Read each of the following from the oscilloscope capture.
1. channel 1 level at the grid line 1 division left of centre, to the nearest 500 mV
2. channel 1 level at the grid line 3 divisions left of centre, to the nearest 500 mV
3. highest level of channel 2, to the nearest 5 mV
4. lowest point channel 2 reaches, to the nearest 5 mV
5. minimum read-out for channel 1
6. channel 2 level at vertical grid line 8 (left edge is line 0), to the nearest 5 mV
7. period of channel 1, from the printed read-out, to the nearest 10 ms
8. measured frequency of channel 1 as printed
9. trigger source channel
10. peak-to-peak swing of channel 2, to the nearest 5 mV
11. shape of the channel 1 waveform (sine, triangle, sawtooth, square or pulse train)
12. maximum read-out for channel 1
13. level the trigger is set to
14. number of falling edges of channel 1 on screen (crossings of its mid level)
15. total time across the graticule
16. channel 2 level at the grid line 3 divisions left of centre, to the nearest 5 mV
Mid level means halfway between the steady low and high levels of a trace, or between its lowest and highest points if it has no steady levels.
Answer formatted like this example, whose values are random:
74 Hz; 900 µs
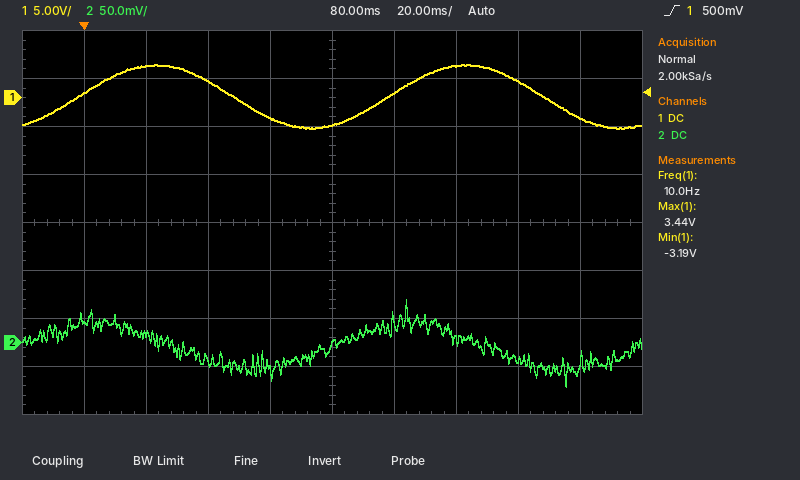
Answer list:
-2.0 V; 3.5 V; 45 mV; -45 mV; -3.19 V; -20 mV; 100 ms; 10.0 Hz; channel 1; 90 mV; sine; 3.44 V; 500 mV; 2; 200 ms; 10 mV
